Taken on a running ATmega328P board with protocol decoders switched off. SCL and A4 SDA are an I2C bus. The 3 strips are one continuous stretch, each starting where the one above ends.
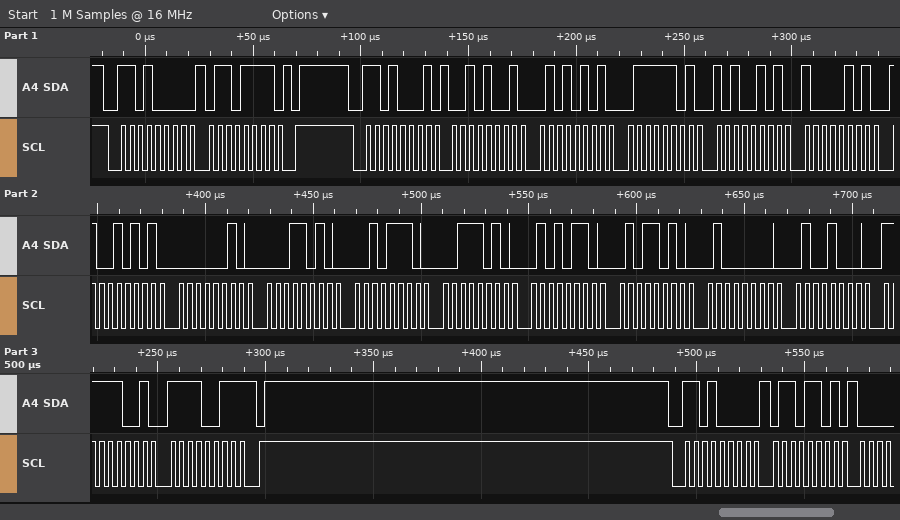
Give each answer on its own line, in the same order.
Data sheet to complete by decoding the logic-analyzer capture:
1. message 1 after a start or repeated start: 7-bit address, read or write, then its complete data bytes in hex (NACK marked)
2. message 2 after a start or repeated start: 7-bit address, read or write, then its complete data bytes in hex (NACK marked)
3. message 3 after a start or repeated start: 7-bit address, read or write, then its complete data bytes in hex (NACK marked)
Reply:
0x68 write: 6F
0x68 read: 29 55 7D A5 85 95 02 1A 2E 3A 56 5A 40 48 F9 F3 NACK
0x68 write: 6D
